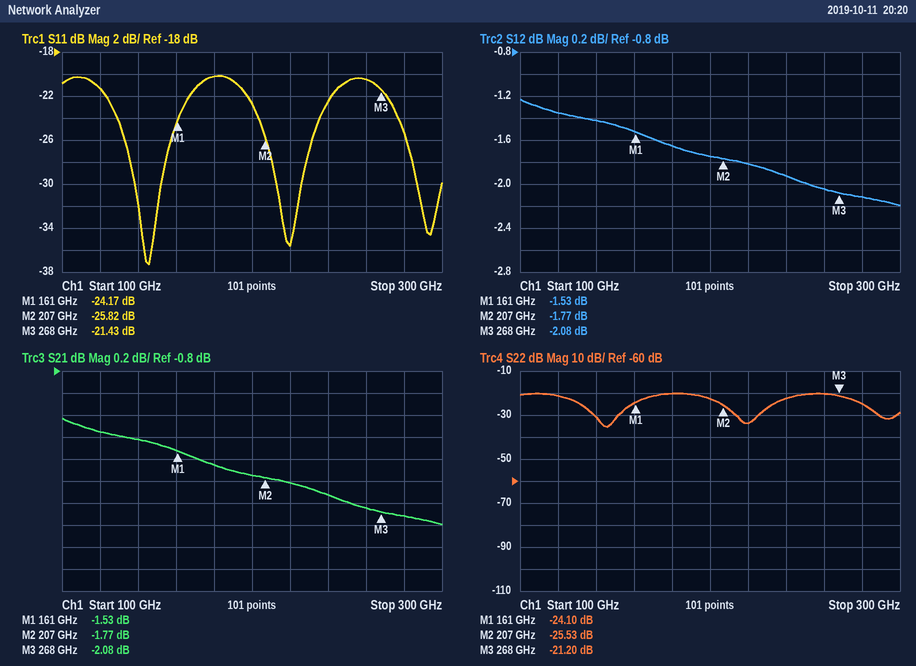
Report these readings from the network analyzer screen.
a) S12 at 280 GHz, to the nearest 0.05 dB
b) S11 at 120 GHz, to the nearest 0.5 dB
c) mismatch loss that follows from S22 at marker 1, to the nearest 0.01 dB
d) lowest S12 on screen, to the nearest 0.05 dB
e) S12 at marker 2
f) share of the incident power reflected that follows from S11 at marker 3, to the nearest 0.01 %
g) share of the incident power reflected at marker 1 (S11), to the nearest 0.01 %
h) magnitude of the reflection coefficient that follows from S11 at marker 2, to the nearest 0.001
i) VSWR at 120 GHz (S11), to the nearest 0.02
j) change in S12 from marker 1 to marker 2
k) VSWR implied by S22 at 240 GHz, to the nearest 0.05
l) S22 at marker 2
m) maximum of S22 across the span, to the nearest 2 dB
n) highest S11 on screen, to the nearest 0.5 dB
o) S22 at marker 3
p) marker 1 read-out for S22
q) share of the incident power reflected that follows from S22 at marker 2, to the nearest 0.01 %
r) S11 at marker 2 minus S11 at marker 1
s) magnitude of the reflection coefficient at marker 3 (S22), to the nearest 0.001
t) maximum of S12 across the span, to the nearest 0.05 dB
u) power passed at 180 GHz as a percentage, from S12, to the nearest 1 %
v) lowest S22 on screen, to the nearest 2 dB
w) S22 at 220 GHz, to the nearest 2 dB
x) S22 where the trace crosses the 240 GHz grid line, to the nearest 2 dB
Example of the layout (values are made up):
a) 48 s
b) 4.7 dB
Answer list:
a) -2.10 dB
b) -21.5 dB
c) 0.02 dB
d) -2.20 dB
e) -1.77 dB
f) 0.72 %
g) 0.38 %
h) 0.051
i) 1.18
j) -0.24 dB
k) 1.15
l) -25.53 dB
m) -20 dB
n) -20.0 dB
o) -21.20 dB
p) -24.10 dB
q) 0.28 %
r) -1.65 dB
s) 0.087
t) -1.25 dB
u) 68 %
v) -36 dB
w) -34 dB
x) -22 dB
